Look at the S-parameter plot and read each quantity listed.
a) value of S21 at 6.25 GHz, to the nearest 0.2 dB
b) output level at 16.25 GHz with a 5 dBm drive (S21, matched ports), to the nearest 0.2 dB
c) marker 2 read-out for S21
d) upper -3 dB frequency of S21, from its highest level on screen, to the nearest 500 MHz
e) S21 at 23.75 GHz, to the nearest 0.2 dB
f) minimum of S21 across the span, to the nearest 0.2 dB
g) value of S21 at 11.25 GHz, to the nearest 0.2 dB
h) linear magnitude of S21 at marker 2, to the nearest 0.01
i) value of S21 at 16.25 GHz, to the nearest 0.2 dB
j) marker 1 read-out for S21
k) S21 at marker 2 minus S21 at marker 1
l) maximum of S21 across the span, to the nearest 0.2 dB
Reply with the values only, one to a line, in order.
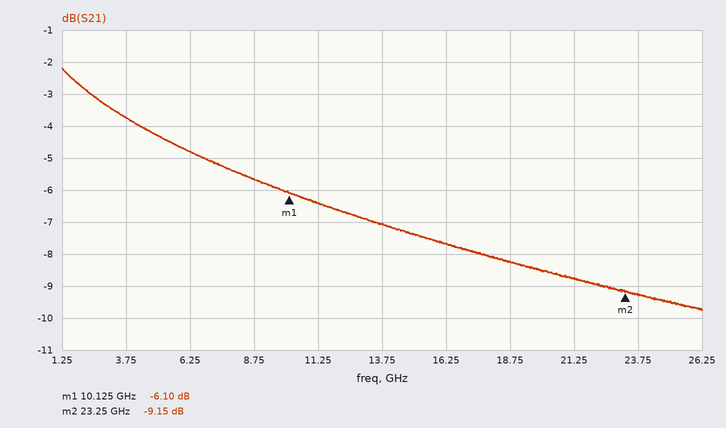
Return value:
-4.8 dB
-2.6 dBm
-9.15 dB
7.5 GHz
-9.2 dB
-9.8 dB
-6.4 dB
0.35
-7.6 dB
-6.10 dB
-3.05 dB
-2.2 dB
